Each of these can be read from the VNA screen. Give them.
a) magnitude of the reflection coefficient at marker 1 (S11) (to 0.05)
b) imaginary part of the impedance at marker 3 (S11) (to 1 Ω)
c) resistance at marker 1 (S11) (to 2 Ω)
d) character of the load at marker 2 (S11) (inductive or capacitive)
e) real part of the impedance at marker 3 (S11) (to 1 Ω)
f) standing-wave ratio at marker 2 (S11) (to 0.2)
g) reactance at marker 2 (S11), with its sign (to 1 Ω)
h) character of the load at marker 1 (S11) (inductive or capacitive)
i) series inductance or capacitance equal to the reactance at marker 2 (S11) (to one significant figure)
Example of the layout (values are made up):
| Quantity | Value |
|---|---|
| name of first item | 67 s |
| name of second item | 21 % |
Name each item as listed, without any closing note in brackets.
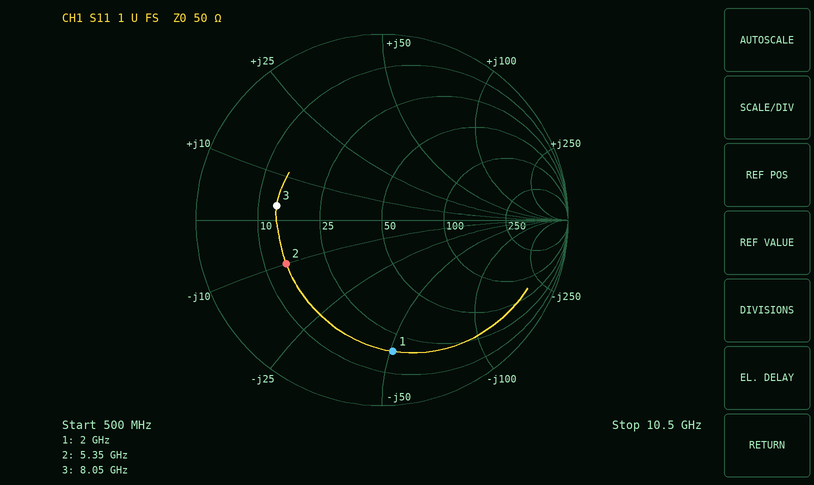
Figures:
| Quantity | Value |
|---|---|
| magnitude of the reflection coefficient at marker 1 (S11) | 0.70 |
| imaginary part of the impedance at marker 3 (S11) | +3 Ω |
| resistance at marker 1 (S11) | 18 Ω |
| character of the load at marker 2 (S11) | capacitive |
| real part of the impedance at marker 3 (S11) | 14 Ω |
| standing-wave ratio at marker 2 (S11) | 3.6 |
| reactance at marker 2 (S11), with its sign | -10 Ω |
| character of the load at marker 1 (S11) | capacitive |
| series inductance or capacitance equal to the reactance at marker 2 (S11) | 3 pF |
